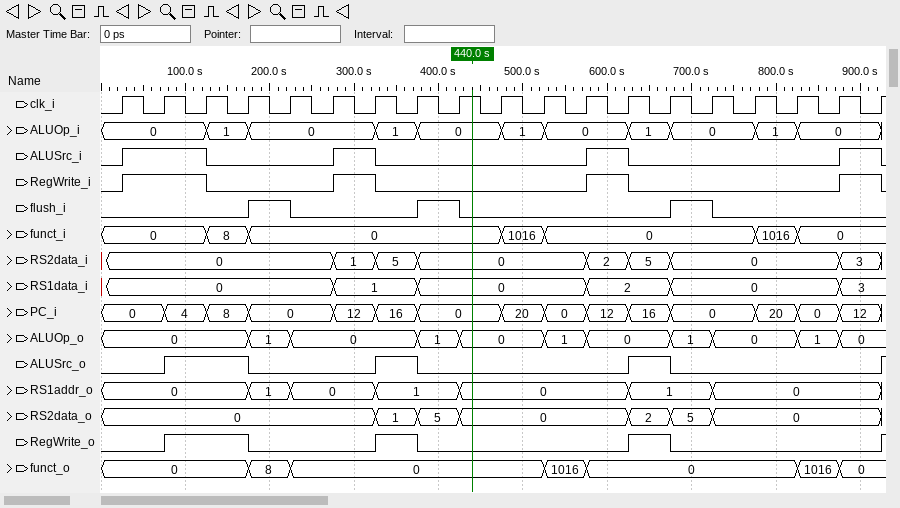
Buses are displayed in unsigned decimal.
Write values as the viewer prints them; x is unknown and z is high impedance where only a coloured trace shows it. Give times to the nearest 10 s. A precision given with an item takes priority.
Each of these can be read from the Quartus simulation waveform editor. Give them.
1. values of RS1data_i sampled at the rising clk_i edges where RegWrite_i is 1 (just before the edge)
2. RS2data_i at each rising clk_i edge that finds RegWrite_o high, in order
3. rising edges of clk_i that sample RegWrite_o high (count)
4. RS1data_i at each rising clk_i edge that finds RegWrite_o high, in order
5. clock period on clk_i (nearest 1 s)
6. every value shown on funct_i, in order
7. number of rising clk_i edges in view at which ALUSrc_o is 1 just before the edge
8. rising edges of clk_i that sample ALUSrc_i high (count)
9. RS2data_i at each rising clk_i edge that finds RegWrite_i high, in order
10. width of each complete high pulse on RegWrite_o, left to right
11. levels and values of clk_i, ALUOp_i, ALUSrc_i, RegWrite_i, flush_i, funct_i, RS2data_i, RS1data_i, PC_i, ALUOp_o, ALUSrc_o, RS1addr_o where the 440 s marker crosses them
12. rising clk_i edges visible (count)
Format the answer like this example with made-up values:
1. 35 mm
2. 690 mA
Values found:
1. 0, 0, 1, 2, 3
2. 0, 0, 5, 5
3. 4
4. 0, 0, 1, 2
5. 50 s
6. 0, 8, 0, 1016, 0, 1016, 0
7. 4
8. 5
9. 0, 0, 1, 2, 3
10. 100 s, 50 s, 50 s
11. clk_i=1, ALUOp_i=0, ALUSrc_i=0, RegWrite_i=0, flush_i=0, funct_i=0, RS2data_i=0, RS1data_i=0, PC_i=0, ALUOp_o=0, ALUSrc_o=0, RS1addr_o=0
12. 19
